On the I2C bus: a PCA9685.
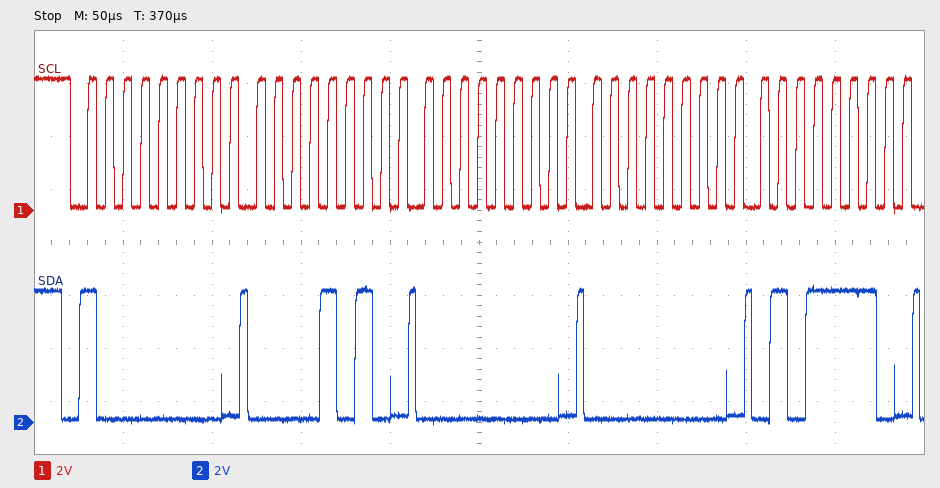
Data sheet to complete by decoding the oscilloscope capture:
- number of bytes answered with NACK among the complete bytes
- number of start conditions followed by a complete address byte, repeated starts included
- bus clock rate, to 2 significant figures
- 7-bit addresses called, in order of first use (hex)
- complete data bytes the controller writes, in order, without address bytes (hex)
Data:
0
1
100 kHz
0x40
0A 00 00 5E
